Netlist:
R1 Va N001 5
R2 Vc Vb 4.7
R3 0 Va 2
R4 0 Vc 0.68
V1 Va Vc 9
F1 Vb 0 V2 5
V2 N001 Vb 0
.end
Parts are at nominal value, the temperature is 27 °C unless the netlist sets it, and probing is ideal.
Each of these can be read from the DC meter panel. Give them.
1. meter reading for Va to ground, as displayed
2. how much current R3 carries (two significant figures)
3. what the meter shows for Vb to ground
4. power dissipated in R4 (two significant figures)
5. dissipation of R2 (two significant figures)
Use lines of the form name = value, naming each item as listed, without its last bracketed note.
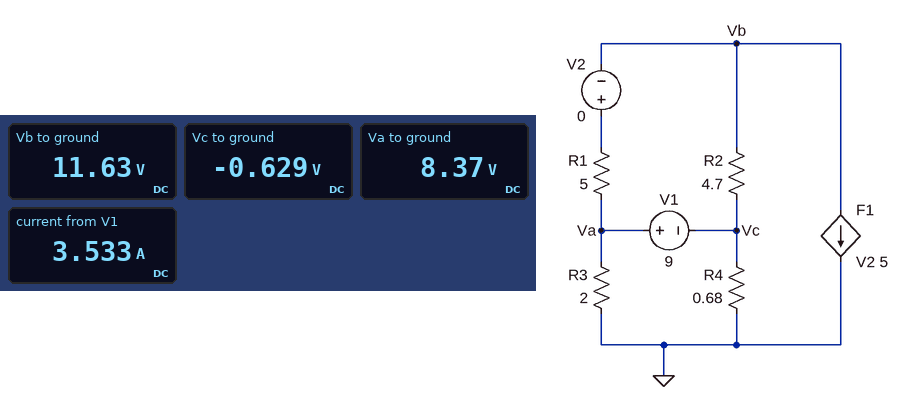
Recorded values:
meter reading for Va to ground, as displayed = 8.37 V
how much current R3 carries = 4.2 A
what the meter shows for Vb to ground = 11.63 V
power dissipated in R4 = 580 mW
dissipation of R2 = 32 W
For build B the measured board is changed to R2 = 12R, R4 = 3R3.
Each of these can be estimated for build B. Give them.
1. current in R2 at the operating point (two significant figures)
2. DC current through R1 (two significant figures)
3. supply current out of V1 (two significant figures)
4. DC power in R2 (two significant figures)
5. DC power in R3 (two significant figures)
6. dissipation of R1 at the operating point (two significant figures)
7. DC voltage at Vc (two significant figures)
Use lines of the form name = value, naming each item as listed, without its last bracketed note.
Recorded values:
current in R2 at the operating point = 840 mA
DC current through R1 = 210 mA
supply current out of V1 = 2.1 A
DC power in R2 = 8.4 W
DC power in R3 = 11 W
dissipation of R1 at the operating point = 220 mW
DC voltage at Vc = -4.3 V
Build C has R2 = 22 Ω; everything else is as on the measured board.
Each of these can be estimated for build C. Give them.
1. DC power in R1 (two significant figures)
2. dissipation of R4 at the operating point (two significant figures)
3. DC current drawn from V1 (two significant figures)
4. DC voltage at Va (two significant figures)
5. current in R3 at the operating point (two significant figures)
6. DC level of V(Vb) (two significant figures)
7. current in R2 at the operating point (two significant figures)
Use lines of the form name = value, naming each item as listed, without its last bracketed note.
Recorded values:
DC power in R1 = 59 mW
dissipation of R4 at the operating point = 5.9 W
DC current drawn from V1 = 3.4 A
DC voltage at Va = 7.0 V
current in R3 at the operating point = 3.5 A
DC level of V(Vb) = 7.5 V
current in R2 at the operating point = 430 mA
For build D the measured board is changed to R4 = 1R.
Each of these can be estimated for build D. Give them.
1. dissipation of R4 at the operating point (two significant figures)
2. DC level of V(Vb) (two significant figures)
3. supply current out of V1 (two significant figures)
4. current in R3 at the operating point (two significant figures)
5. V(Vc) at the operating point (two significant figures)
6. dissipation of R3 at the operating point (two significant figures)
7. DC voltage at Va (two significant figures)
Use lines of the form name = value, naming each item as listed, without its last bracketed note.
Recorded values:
dissipation of R4 at the operating point = 680 mW
DC level of V(Vb) = 11 V
supply current out of V1 = 3.4 A
current in R3 at the operating point = 4.1 A
V(Vc) at the operating point = -830 mV
dissipation of R3 at the operating point = 33 W
DC voltage at Va = 8.2 V
